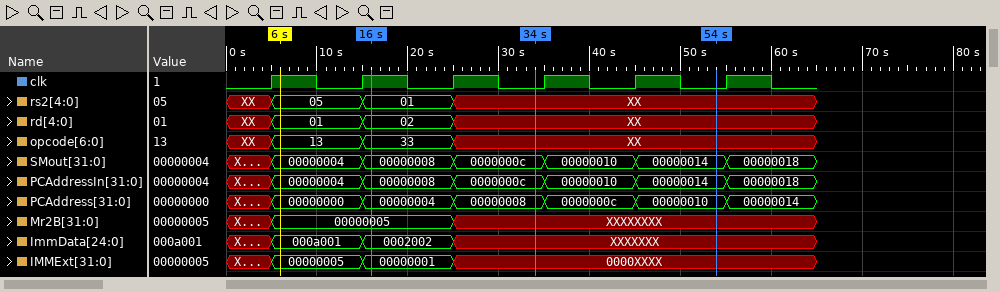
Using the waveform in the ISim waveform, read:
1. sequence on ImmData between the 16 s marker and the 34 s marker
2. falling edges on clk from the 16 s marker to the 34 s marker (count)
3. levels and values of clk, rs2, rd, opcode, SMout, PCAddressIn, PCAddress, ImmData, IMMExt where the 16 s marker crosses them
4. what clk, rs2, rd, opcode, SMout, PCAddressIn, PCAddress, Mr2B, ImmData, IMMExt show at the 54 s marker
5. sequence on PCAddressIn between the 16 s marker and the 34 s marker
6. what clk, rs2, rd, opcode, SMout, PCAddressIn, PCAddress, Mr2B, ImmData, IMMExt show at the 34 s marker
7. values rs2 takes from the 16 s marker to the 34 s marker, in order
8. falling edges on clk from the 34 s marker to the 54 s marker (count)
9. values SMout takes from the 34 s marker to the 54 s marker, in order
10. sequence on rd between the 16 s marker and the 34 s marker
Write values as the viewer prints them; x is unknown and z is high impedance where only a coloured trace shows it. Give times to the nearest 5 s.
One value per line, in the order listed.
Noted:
0002002, XXXXXXX
2
clk=1, rs2=01, rd=02, opcode=33, SMout=00000008, PCAddressIn=00000008, PCAddress=00000004, ImmData=0002002, IMMExt=00000001
clk=0, rs2=XX, rd=XX, opcode=XX, SMout=00000014, PCAddressIn=00000014, PCAddress=00000010, Mr2B=XXXXXXXX, ImmData=XXXXXXX, IMMExt=0000XXXX
00000008, 0000000c
clk=0, rs2=XX, rd=XX, opcode=XX, SMout=0000000c, PCAddressIn=0000000c, PCAddress=00000008, Mr2B=XXXXXXXX, ImmData=XXXXXXX, IMMExt=0000XXXX
01, XX
2
0000000c, 00000010, 00000014
02, XX
